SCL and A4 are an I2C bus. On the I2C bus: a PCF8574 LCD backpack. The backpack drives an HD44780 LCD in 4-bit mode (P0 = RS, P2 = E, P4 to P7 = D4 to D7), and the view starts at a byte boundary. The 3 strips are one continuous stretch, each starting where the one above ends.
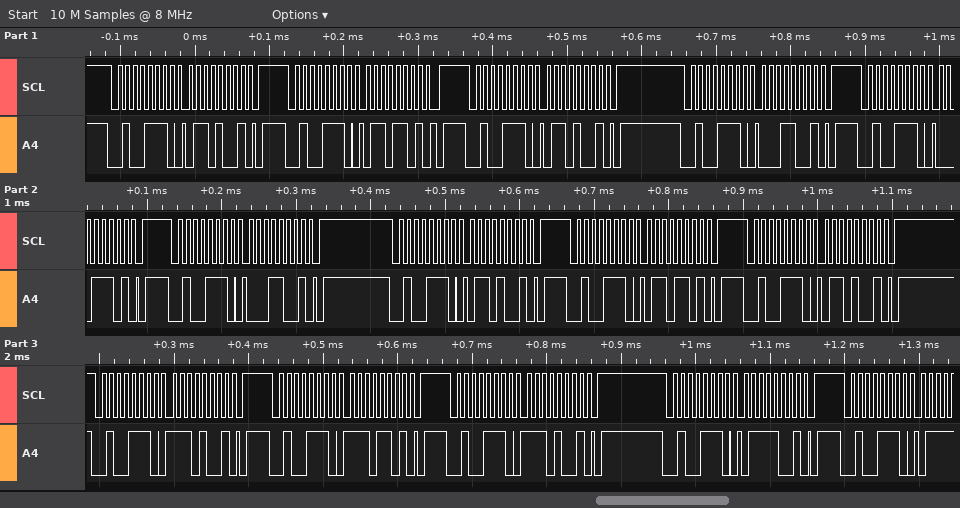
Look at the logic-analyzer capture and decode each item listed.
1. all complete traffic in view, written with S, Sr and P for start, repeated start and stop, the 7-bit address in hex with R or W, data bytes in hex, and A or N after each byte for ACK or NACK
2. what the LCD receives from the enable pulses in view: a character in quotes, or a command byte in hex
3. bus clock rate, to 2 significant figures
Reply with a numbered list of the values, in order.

1. S 27W A 69 A P S 27W A 6D A P S 27W A 69 A P S 27W A 19 A P S 27W A 1D A P S 27W A 19 A P S 27W A 69 A P S 27W A 6D A P S 27W A 69 A P S 27W A E9 A P S 27W A ED A P S 27W A E9 A P S 27W A 79 A P S 27W A
2. 'a' 'n'
3. 100 kHz
